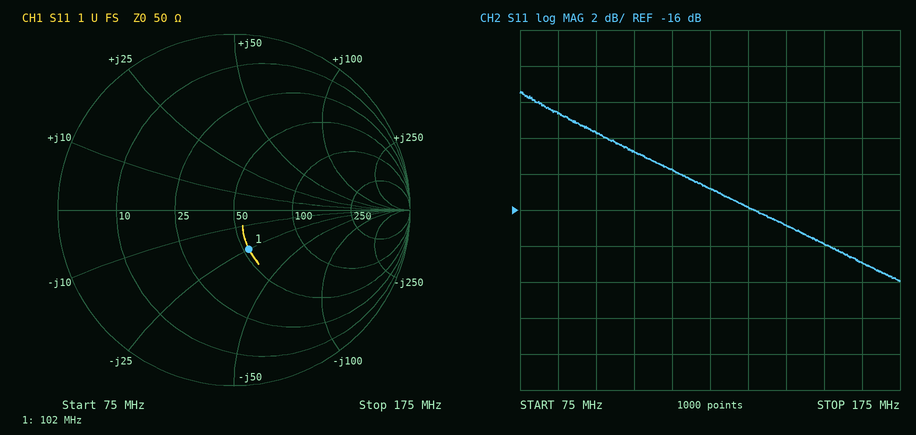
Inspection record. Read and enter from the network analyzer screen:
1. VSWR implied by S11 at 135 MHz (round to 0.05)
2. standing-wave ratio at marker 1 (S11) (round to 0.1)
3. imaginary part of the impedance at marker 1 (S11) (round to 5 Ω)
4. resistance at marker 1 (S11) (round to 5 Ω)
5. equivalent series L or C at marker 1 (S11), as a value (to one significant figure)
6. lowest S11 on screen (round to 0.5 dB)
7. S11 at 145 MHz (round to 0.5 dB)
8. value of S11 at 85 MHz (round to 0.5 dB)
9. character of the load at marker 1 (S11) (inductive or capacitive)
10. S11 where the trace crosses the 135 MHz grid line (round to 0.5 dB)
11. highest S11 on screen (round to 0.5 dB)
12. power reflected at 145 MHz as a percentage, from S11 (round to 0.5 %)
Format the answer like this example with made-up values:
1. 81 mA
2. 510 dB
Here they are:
1. 1.40
2. 1.6
3. -25 Ω
4. 55 Ω
5. 60 pF
6. -20.0 dB
7. -17.0 dB
8. -10.5 dB
9. capacitive
10. -16.0 dB
11. -9.5 dB
12. 2.0 %
